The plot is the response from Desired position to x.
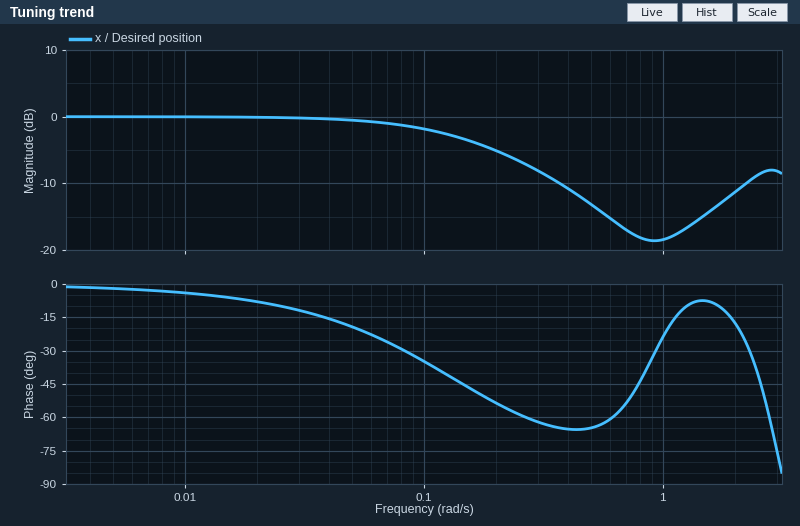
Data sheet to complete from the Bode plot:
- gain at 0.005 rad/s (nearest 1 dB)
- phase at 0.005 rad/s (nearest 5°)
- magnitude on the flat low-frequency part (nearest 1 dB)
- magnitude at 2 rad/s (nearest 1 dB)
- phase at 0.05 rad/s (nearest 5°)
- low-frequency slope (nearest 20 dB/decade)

0 dB
0°
0 dB
-11 dB
-20°
0 dB/decade
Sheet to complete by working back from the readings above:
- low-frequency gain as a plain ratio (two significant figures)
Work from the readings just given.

1.0
